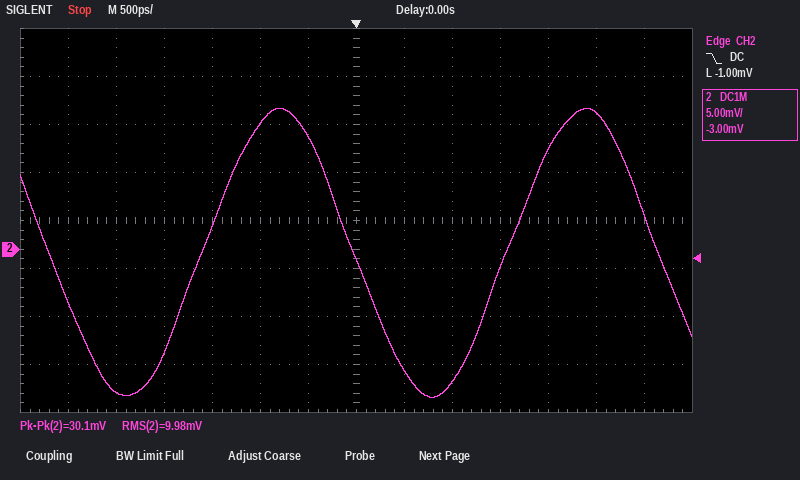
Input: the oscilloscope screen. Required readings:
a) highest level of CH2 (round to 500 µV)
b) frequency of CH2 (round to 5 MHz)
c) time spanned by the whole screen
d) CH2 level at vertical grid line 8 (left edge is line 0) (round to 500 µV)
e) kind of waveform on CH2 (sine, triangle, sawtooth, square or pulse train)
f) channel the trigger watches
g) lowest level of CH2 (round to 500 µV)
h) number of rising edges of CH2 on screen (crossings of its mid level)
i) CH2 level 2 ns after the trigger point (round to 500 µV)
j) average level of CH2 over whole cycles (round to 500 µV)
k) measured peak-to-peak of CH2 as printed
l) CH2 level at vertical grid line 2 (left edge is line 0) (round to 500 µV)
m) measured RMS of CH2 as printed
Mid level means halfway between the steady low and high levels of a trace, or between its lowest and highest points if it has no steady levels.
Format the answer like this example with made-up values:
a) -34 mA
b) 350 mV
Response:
a) 14.5 mV
b) 315 MHz
c) 7 ns
d) -12.5 mV
e) sine
f) CH2
g) -15.5 mV
h) 2
i) 10.5 mV
j) -500 µV
k) 30.1 mV
l) -15.0 mV
m) 9.98 mV
